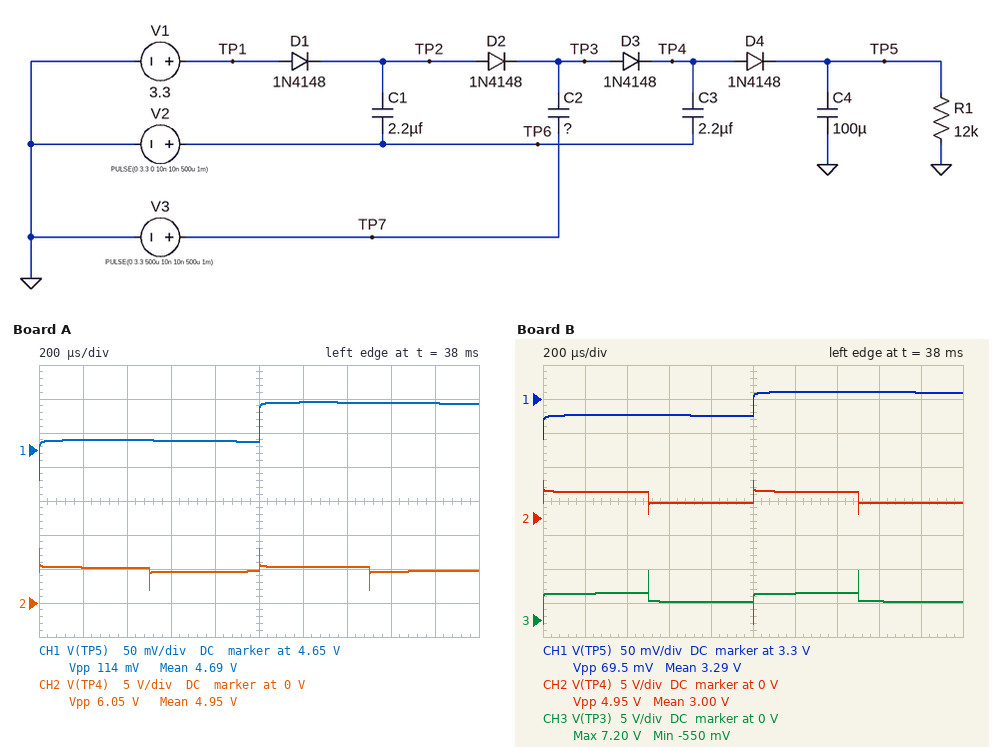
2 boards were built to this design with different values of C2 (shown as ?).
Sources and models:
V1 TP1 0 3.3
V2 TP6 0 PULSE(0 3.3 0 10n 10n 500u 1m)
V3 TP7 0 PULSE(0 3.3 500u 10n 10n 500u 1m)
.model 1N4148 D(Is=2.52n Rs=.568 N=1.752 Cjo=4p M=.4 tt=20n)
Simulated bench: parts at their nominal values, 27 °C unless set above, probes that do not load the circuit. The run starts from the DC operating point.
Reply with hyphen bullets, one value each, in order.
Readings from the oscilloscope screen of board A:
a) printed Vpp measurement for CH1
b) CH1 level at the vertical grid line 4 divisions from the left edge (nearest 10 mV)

- 114 mV
- 4.66 V
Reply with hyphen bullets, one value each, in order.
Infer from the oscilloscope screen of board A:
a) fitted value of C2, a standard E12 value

- 6.8 µF
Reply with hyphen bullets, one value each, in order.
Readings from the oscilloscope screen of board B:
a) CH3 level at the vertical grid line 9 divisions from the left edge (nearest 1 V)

- 3 V
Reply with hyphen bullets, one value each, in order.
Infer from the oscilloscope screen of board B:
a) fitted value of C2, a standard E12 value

- 820 nF
